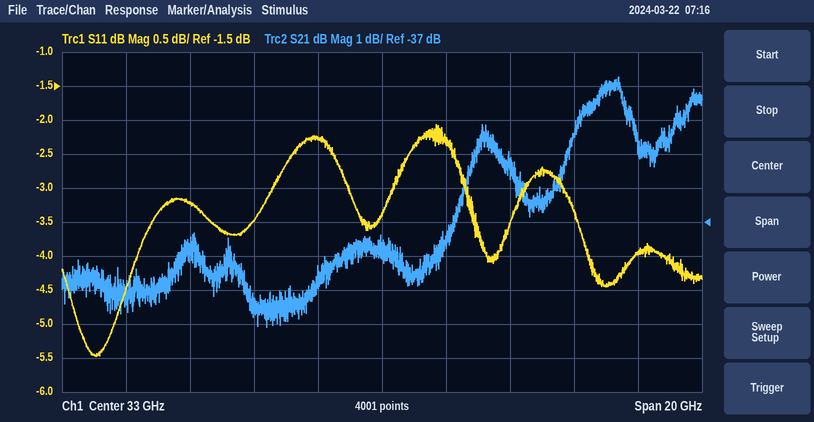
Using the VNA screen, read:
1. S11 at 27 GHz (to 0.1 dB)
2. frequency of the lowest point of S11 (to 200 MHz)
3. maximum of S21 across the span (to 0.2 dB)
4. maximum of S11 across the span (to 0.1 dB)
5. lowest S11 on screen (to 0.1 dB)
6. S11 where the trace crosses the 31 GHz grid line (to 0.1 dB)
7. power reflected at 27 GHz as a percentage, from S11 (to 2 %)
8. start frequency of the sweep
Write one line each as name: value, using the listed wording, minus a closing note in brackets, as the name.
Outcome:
S11 at 27 GHz: -3.2 dB
frequency of the lowest point of S11: 24.0 GHz
maximum of S21 across the span: -32.8 dB
maximum of S11 across the span: -2.1 dB
lowest S11 on screen: -5.5 dB
S11 where the trace crosses the 31 GHz grid line: -2.3 dB
power reflected at 27 GHz as a percentage, from S11: 48 %
start frequency of the sweep: 23 GHz
